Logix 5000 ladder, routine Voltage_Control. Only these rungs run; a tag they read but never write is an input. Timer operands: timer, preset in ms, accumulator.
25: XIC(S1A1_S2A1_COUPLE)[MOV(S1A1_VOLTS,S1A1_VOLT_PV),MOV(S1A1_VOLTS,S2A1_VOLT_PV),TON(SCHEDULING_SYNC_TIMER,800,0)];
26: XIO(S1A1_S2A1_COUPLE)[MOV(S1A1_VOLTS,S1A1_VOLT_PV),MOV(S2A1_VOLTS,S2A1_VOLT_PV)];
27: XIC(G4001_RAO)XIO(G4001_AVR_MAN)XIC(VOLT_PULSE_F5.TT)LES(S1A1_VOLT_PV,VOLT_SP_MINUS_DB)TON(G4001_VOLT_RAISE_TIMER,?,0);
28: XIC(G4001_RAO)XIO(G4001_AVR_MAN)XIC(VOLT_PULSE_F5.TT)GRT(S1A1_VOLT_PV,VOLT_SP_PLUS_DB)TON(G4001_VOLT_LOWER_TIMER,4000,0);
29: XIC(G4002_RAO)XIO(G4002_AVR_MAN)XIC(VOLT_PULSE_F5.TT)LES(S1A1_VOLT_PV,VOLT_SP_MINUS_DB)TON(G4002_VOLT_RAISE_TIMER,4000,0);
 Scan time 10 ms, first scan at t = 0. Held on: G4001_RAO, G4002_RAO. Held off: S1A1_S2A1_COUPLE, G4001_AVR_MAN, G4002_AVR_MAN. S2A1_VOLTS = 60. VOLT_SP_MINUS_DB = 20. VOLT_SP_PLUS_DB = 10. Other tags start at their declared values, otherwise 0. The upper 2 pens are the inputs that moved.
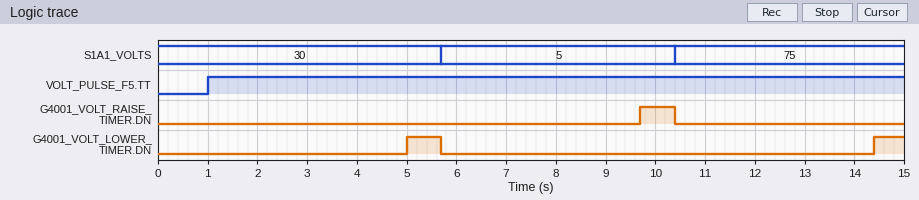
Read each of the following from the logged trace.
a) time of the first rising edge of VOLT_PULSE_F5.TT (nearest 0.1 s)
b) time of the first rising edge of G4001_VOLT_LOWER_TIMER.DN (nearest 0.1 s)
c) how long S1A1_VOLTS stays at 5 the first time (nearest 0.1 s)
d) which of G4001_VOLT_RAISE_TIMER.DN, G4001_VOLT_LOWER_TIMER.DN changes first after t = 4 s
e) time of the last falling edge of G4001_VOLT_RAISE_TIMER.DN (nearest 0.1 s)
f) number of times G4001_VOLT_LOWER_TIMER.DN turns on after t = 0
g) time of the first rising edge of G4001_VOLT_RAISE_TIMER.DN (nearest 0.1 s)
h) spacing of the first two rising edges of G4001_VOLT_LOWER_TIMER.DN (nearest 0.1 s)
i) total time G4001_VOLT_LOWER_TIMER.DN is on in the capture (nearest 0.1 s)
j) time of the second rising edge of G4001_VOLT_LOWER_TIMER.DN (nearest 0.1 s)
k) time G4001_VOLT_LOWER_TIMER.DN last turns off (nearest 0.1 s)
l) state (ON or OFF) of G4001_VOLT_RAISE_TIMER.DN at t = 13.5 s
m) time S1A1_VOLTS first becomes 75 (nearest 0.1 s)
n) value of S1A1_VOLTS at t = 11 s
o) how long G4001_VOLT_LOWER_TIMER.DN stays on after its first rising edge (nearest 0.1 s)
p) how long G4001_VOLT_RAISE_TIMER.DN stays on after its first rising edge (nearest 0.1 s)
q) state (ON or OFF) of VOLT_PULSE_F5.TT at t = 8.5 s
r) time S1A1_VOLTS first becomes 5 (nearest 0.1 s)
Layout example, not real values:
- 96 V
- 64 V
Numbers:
- 1.0 s
- 5.0 s
- 4.7 s
- G4001_VOLT_LOWER_TIMER.DN
- 10.4 s
- 2
- 9.7 s
- 9.4 s
- 1.3 s
- 14.4 s
- 5.7 s
- OFF
- 10.4 s
- 75
- 0.7 s
- 0.7 s
- ON
- 5.7 s
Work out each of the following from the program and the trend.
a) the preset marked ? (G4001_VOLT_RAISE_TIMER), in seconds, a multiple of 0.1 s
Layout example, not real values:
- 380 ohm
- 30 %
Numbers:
- 4.0 s
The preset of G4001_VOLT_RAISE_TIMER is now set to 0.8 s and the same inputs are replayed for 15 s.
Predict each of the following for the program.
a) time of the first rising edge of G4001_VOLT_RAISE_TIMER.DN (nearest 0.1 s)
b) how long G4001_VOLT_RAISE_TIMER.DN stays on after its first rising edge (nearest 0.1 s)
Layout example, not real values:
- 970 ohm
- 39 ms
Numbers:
- 6.5 s
- 3.9 s
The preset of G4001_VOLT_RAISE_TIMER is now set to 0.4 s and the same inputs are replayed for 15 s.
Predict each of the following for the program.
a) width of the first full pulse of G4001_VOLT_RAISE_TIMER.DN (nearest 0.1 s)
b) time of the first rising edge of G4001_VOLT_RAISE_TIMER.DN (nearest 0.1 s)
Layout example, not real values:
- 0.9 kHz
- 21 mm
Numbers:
- 4.3 s
- 6.1 s
